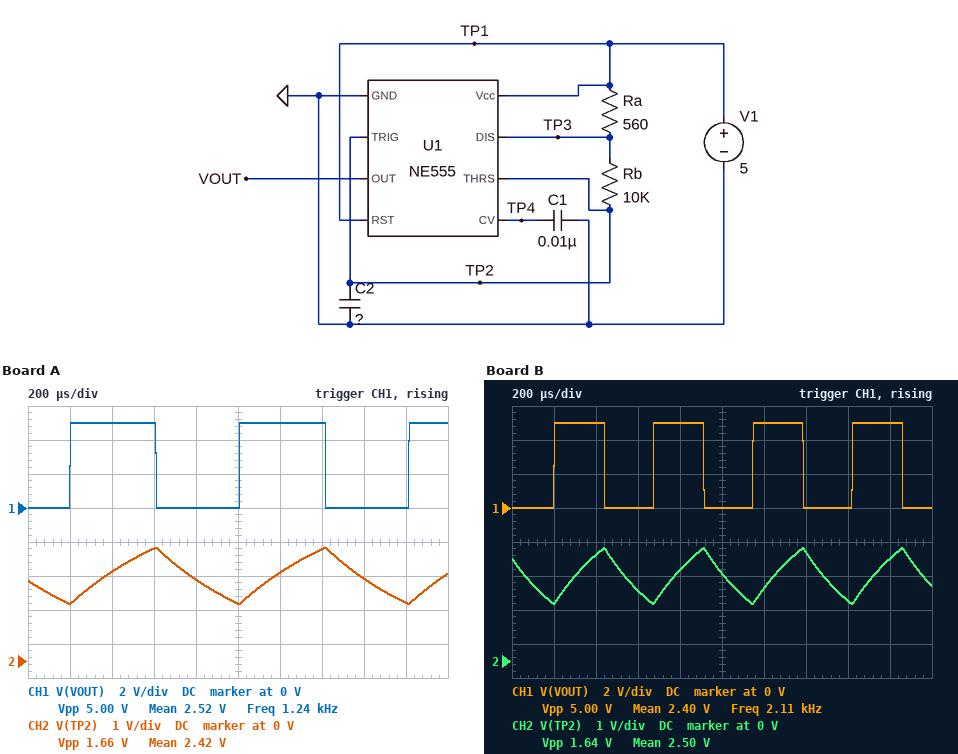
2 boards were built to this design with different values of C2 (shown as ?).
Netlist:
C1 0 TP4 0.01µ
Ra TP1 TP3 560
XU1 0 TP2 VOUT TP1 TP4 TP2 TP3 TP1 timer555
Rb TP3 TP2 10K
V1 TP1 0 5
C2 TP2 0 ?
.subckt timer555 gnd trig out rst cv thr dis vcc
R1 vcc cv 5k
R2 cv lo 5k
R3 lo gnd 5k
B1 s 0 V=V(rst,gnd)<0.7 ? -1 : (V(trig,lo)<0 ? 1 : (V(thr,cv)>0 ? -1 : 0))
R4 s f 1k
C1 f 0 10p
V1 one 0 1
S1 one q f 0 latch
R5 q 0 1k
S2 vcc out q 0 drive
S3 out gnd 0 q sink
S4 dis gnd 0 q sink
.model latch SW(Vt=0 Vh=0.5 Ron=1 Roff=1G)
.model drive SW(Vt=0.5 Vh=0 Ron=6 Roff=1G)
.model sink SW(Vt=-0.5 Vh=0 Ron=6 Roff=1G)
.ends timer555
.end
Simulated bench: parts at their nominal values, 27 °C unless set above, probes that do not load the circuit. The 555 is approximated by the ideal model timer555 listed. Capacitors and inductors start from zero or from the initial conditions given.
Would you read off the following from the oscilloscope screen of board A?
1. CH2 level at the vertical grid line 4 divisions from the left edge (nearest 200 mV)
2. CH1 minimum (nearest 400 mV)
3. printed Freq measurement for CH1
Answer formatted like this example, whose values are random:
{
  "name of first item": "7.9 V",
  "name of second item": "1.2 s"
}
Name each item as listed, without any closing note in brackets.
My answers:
{
  "CH2 level at the vertical grid line 4 divisions from the left edge": "2.4 V",
  "CH1 minimum": "0 V",
  "printed Freq measurement for CH1": "1.24 kHz"
}
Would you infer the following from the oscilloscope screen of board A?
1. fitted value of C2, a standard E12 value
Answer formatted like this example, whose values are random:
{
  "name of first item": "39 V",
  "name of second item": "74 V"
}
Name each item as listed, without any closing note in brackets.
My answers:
{
  "fitted value of C2, a standard E12 value": "56 nF"
}
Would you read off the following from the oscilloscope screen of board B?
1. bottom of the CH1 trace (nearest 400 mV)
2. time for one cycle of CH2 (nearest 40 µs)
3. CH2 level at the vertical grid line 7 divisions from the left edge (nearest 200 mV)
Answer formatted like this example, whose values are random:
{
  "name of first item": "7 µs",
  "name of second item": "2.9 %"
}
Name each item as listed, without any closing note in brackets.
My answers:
{
  "bottom of the CH1 trace": "0 V",
  "time for one cycle of CH2": "480 µs",
  "CH2 level at the vertical grid line 7 divisions from the left edge": "3.2 V"
}
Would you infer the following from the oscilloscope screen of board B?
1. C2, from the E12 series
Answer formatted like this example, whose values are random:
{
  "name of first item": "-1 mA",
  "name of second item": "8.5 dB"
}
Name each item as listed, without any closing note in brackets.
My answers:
{
  "C2, from the E12 series": "33 nF"
}
